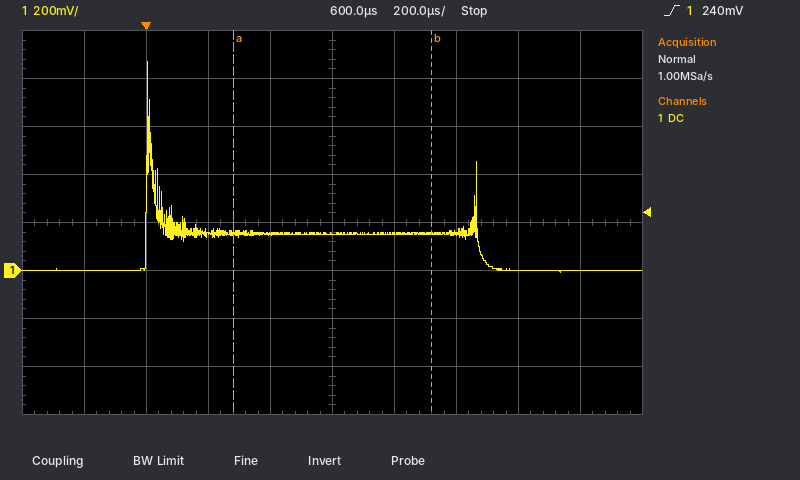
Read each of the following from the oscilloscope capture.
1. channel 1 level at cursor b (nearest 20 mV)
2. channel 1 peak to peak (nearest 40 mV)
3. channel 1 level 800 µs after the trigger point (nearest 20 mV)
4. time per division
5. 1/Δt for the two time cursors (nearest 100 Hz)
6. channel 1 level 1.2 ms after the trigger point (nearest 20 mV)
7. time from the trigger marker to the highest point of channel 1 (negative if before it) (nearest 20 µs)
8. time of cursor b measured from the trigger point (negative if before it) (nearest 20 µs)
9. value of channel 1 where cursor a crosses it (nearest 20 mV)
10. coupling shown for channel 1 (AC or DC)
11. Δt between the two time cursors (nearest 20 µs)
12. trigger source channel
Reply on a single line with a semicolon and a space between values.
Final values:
160 mV; 880 mV; 160 mV; 200 µs; 1.6 kHz; 0 mV; 0 µs; +920 µs; 160 mV; DC; 640 µs; channel 1
